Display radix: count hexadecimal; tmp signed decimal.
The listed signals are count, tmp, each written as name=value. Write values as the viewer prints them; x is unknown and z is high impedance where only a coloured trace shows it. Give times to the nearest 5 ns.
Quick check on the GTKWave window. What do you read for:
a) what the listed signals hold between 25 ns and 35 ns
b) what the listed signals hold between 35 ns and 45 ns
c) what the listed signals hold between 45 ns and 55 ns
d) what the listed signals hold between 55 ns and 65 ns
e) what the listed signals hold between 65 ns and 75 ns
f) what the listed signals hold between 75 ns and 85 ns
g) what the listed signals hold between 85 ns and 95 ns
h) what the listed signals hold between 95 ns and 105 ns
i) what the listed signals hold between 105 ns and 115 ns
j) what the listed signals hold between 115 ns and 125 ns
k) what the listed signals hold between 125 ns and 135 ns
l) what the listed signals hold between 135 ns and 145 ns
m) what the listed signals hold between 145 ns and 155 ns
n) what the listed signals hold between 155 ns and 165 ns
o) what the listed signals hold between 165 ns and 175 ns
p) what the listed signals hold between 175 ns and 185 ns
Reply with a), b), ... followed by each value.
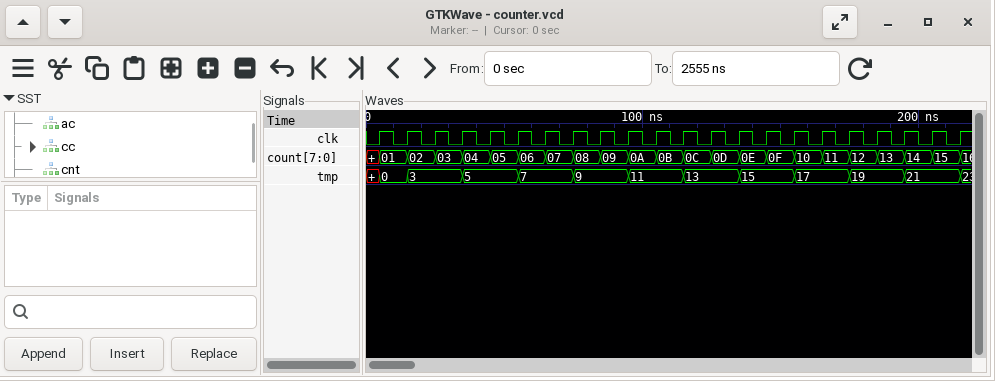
a) count=03, tmp=3
b) count=04, tmp=5
c) count=05, tmp=5
d) count=06, tmp=7
e) count=07, tmp=7
f) count=08, tmp=9
g) count=09, tmp=9
h) count=0A, tmp=11
i) count=0B, tmp=11
j) count=0C, tmp=13
k) count=0D, tmp=13
l) count=0E, tmp=15
m) count=0F, tmp=15
n) count=10, tmp=17
o) count=11, tmp=17
p) count=12, tmp=19
